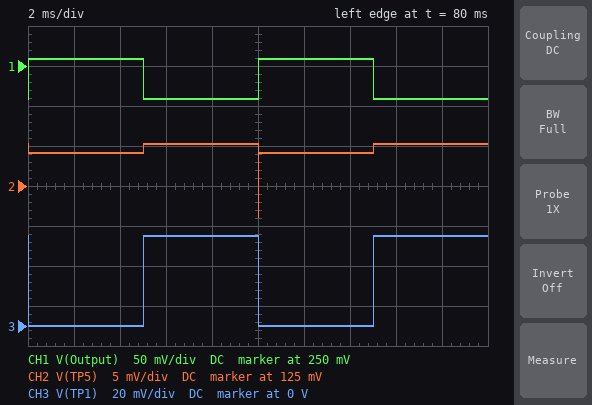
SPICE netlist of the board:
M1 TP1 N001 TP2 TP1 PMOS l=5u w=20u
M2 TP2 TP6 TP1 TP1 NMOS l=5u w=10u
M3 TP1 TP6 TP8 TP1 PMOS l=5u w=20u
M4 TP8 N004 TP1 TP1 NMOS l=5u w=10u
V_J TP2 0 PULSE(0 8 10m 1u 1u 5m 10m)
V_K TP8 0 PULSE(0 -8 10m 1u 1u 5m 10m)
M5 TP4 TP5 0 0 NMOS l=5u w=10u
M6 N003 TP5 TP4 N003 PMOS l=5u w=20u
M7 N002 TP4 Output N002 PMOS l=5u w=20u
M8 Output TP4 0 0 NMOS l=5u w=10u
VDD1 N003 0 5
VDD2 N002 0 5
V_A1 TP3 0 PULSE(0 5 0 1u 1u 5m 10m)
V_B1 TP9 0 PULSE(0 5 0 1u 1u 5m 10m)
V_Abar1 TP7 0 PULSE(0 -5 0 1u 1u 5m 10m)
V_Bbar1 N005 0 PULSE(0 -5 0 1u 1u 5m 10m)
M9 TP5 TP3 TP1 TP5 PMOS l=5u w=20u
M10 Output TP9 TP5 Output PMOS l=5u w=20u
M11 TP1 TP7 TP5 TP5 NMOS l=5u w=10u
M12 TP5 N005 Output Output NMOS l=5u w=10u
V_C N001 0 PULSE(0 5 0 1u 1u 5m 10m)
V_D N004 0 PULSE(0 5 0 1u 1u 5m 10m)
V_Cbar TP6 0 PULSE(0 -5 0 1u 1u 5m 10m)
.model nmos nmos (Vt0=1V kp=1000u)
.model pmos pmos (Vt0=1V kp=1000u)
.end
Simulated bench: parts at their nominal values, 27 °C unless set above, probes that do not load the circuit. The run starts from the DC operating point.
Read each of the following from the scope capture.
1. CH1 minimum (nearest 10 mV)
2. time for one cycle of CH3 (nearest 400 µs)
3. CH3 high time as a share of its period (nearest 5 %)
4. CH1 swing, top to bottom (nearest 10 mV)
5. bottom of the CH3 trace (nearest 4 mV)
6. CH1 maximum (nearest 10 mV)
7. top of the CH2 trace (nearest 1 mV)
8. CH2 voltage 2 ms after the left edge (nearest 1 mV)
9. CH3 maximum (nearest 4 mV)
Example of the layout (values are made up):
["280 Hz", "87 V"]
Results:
["210 mV", "10.0 ms", "50 %", "50 mV", "0 V", "260 mV", "130 mV", "129 mV", "44 mV"]
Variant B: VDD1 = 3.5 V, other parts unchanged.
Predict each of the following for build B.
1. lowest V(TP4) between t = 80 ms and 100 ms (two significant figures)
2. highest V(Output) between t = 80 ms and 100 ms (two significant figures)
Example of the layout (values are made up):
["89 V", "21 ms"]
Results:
["3.5 V", "1.9 V"]
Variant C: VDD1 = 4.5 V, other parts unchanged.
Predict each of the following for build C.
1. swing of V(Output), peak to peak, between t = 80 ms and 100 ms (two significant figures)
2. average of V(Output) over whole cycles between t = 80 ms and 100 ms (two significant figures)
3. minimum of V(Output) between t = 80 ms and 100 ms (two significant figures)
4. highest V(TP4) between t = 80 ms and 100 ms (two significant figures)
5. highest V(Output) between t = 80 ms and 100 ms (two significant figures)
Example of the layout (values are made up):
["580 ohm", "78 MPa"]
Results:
["190 mV", "620 mV", "530 mV", "4.5 V", "720 mV"]
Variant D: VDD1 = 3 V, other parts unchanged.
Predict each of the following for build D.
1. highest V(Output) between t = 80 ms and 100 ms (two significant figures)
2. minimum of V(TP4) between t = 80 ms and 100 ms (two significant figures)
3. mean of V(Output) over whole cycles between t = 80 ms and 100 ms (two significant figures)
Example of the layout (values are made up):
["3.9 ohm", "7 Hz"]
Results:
["2.1 V", "3.0 V", "1.8 V"]
